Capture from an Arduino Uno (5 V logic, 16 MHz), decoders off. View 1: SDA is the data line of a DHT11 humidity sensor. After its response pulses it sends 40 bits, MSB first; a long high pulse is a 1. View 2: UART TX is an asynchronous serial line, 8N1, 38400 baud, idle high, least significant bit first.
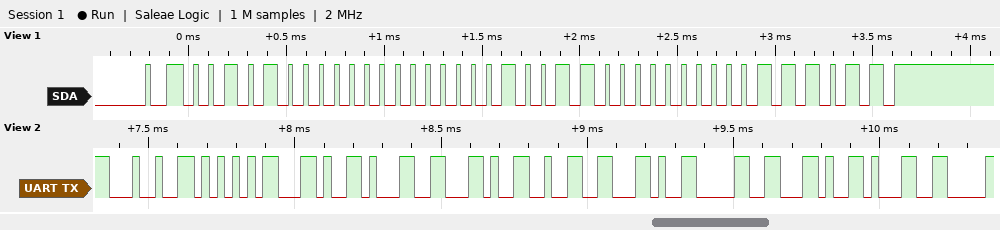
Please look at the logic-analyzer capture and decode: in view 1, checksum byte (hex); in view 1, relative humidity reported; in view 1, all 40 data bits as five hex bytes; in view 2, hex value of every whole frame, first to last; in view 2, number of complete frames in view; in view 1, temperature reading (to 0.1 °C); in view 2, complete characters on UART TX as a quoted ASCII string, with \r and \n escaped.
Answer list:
0x3B
40 %
28 00 13 00 3B
24 55 2C 31 2C 32 2C 30 2C 31
10
19.0 °C
"$U,1,2,0,1"
